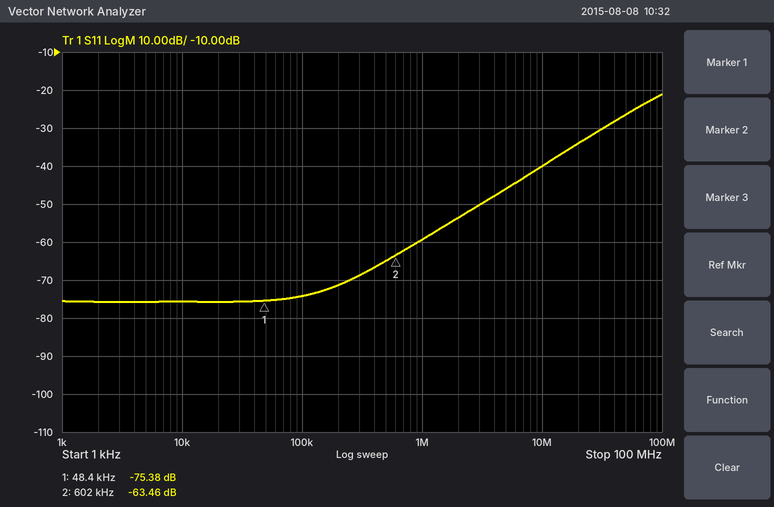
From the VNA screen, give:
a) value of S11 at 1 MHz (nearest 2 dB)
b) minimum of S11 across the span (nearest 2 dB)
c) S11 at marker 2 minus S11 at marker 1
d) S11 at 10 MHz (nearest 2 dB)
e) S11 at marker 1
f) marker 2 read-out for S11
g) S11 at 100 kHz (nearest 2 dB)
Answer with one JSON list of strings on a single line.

["-60 dB", "-76 dB", "11.92 dB", "-40 dB", "-75.38 dB", "-63.46 dB", "-74 dB"]
